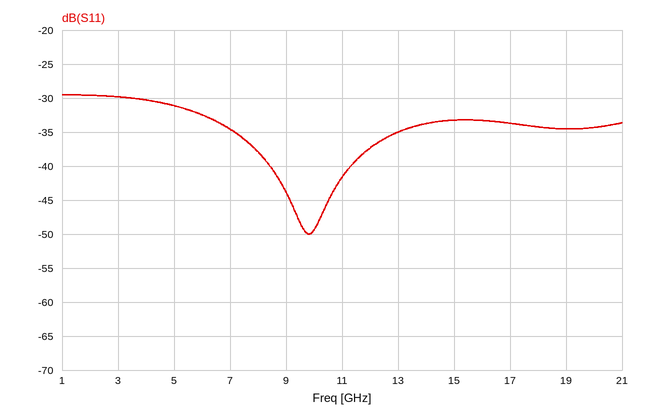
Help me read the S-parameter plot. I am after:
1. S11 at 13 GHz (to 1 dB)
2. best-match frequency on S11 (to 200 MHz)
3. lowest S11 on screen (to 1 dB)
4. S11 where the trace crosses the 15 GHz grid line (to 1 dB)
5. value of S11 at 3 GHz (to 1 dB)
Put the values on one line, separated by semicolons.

-35 dB; 9.8 GHz; -50 dB; -33 dB; -30 dB
